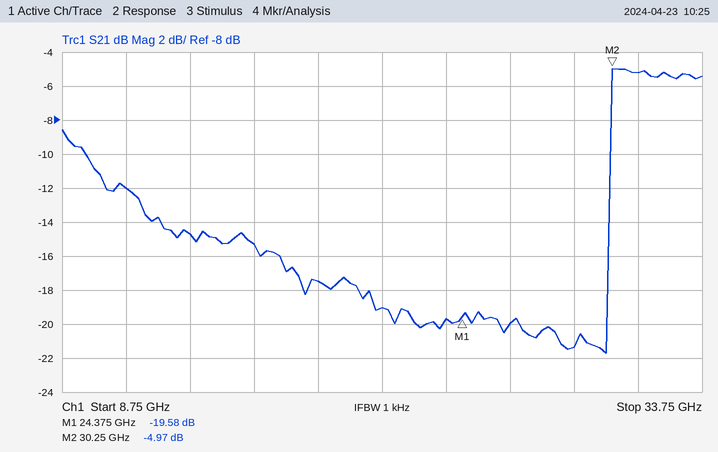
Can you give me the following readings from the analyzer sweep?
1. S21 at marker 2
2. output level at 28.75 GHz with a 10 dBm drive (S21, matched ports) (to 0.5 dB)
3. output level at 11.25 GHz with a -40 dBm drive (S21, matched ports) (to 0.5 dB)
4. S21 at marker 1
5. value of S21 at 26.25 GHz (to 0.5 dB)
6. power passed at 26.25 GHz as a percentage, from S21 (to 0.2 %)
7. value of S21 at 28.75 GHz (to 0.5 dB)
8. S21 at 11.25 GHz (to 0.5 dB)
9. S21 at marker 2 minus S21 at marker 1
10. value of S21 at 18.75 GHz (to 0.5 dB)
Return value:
-4.97 dB
-11.5 dBm
-52.0 dBm
-19.58 dB
-20.0 dB
1.0 %
-21.5 dB
-12.0 dB
14.61 dB
-17.5 dB
